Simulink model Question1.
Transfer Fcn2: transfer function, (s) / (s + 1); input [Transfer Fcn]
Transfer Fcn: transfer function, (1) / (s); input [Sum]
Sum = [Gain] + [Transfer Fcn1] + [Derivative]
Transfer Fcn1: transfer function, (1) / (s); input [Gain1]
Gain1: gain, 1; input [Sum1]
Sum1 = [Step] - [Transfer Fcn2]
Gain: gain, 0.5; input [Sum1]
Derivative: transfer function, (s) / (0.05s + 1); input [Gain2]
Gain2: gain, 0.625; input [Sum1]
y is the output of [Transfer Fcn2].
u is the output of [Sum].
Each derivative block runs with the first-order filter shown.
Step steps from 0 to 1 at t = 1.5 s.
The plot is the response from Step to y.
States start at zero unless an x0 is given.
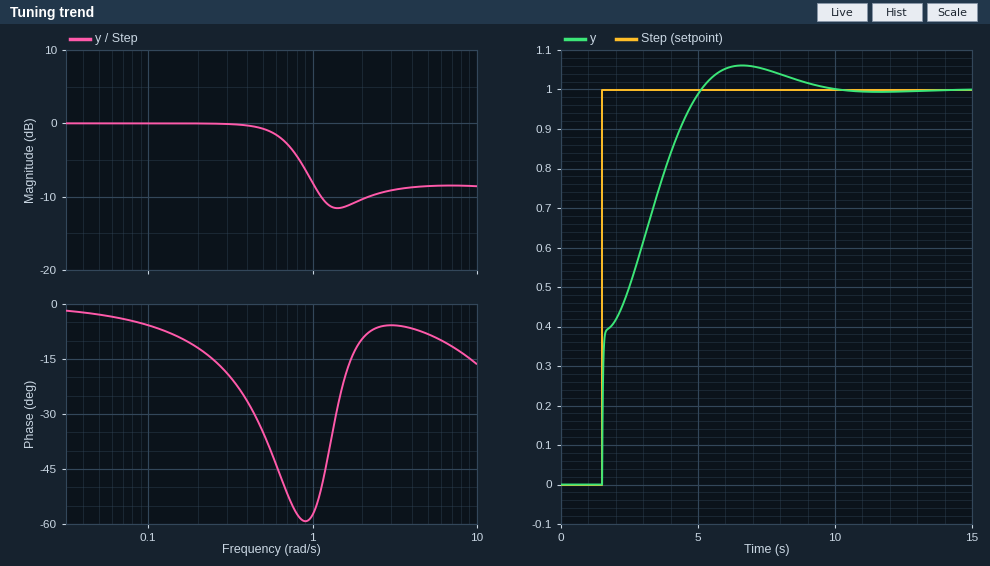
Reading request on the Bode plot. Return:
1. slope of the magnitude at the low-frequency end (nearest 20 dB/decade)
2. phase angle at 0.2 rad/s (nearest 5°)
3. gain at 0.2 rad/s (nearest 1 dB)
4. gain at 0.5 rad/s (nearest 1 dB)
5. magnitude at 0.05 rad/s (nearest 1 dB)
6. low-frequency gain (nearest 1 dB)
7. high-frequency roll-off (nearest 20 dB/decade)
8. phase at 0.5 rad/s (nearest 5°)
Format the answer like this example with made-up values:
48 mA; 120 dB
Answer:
0 dB/decade; -10°; 0 dB; -1 dB; 0 dB; 0 dB; 0 dB/decade; -35°
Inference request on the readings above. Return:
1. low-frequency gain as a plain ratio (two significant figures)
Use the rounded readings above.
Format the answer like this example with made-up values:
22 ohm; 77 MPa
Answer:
1.0
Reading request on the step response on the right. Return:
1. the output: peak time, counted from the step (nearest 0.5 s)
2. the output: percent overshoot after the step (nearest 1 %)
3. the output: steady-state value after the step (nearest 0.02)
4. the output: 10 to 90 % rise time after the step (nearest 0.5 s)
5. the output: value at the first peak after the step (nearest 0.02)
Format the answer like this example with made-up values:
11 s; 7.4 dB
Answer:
5.0 s; 6 %; 1.00; 3.0 s; 1.06
